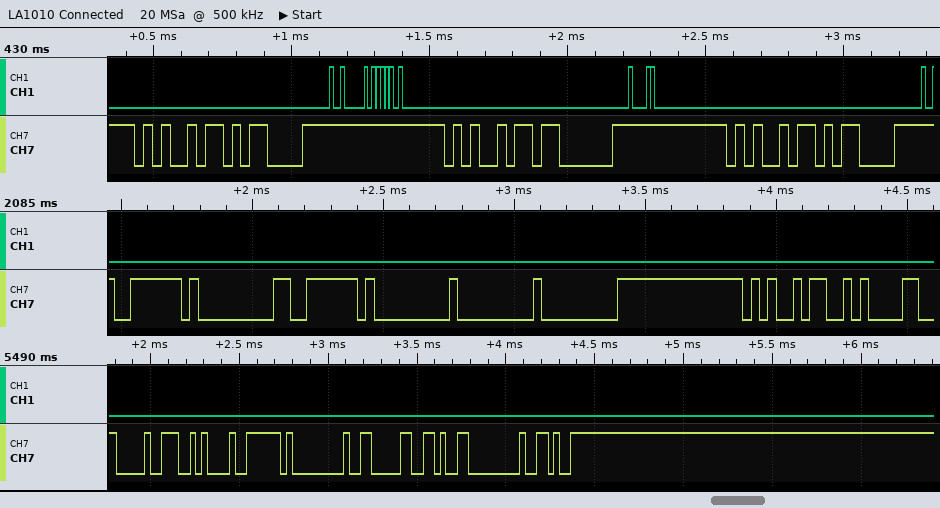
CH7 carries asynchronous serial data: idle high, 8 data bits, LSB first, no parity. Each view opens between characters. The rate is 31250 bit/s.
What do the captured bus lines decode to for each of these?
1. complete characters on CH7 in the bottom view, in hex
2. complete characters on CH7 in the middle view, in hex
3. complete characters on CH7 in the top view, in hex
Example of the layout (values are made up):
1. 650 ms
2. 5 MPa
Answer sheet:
1. 90, 0A, 7E, 00, 06, 96, 00, 96
2. 7E, 00, 7E, 00, 00, 00, A5, 0A
3. A5, 0D, A5, 03, A5, 0D
